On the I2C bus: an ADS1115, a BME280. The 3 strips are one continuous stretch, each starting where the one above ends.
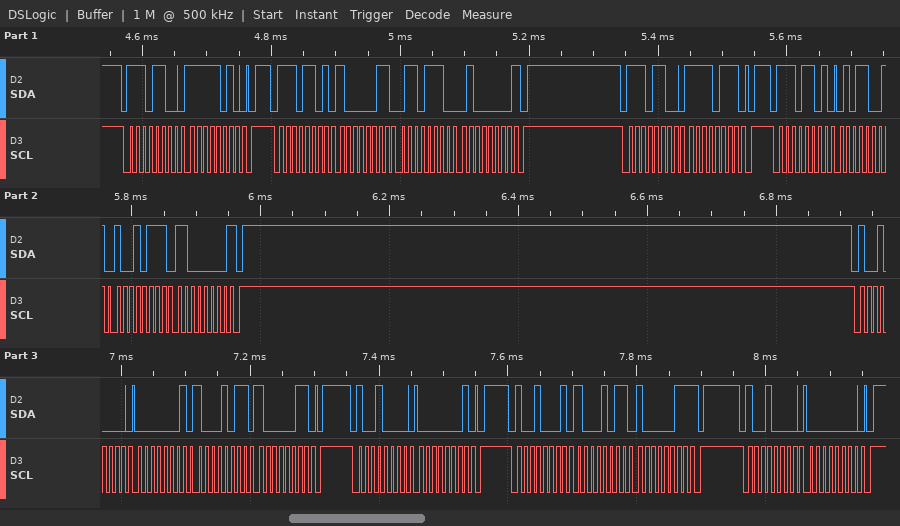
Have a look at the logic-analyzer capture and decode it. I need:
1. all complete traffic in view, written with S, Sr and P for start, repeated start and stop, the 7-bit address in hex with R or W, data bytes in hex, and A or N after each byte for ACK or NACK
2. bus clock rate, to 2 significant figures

S 76W A FA A P S 76R A 83 A 6E A 40 N P S 76W A F7 A P S 76R A 59 A 97 A C0 N P S 48W A 01 A 8B A 83 A P S 48W A 01 A P S 48R A 8B A 83 N P S 48W A 00 A P
100 kHz
